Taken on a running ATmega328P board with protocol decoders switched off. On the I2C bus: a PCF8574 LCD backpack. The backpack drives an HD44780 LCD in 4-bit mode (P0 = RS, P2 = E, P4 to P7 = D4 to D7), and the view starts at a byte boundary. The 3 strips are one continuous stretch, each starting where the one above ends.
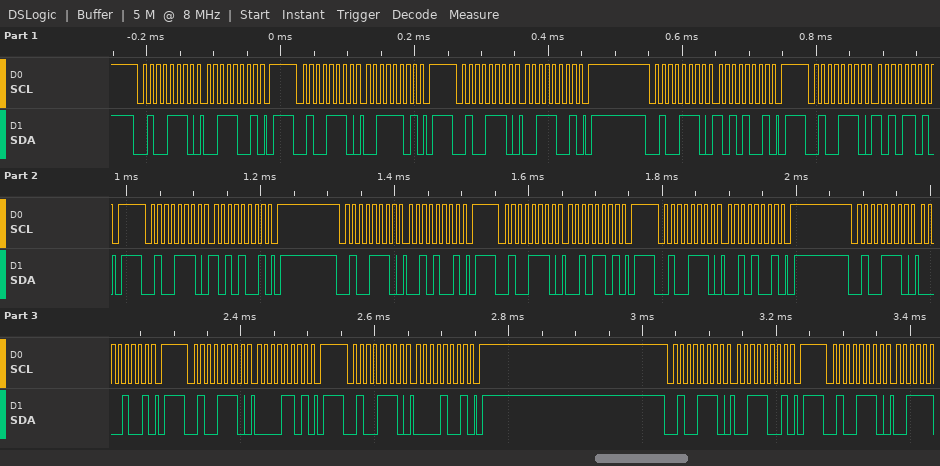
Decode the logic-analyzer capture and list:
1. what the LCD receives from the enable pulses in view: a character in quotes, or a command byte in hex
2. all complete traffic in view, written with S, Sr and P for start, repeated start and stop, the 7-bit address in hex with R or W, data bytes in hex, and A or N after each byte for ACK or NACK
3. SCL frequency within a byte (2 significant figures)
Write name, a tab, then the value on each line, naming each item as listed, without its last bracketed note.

what the LCD receives from the enable pulses in view: a character in quotes, or a command byte in hex	':' ' '
all complete traffic in view, written with S, Sr and P for start, repeated start and stop, the 7-bit address in hex with R or W, data bytes in hex, and A or N after each byte for ACK or NACK	S 27W A 39 A P S 27W A 3D A P S 27W A 39 A P S 27W A A9 A P S 27W A AD A P S 27W A A9 A P S 27W A 29 A P S 27W A 2D A P S 27W A 29 A P S 27W A 09 A P S 27W A 0D A P S 27W A 09 A P S 27W A 39 A P S 27W A
SCL frequency within a byte	100 kHz
